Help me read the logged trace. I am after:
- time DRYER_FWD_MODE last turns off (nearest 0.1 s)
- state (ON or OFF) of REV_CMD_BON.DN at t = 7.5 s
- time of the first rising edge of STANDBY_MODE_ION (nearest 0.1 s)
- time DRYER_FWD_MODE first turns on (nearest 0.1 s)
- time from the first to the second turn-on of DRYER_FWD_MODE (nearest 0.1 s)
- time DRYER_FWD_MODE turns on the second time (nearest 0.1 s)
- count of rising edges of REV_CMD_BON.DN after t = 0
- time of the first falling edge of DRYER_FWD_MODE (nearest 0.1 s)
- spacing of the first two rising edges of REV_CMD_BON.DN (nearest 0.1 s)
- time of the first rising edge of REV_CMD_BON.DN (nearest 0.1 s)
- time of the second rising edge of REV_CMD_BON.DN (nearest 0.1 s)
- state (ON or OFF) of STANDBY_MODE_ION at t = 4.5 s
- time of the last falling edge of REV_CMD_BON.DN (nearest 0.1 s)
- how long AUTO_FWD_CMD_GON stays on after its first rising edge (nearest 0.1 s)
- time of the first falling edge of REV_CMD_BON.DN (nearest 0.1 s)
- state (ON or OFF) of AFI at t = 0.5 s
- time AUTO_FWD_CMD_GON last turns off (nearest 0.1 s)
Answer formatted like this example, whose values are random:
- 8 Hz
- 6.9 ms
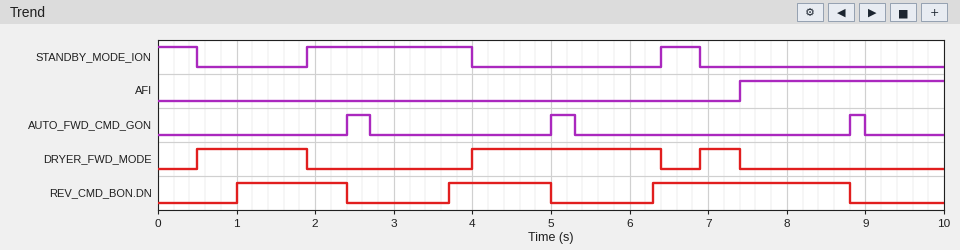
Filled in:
- 7.4 s
- ON
- 1.9 s
- 0.5 s
- 3.5 s
- 4.0 s
- 3
- 1.9 s
- 2.7 s
- 1.0 s
- 3.7 s
- OFF
- 8.8 s
- 0.3 s
- 2.4 s
- OFF
- 9.0 s
